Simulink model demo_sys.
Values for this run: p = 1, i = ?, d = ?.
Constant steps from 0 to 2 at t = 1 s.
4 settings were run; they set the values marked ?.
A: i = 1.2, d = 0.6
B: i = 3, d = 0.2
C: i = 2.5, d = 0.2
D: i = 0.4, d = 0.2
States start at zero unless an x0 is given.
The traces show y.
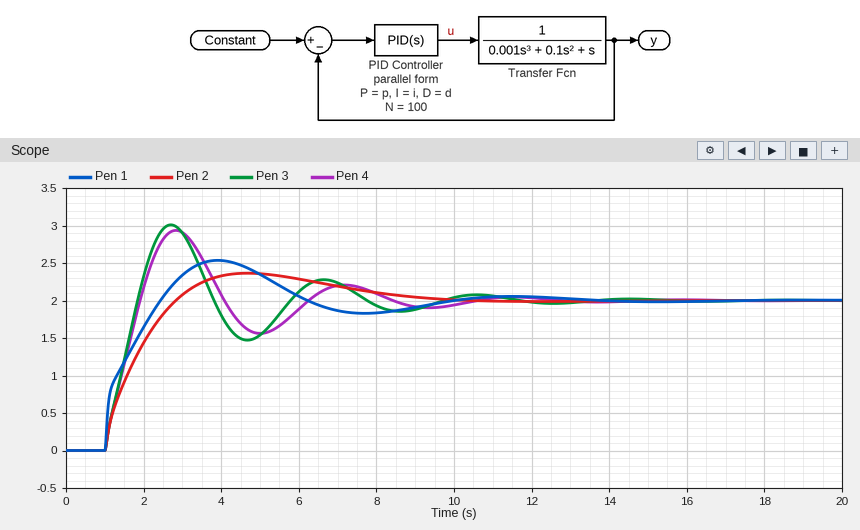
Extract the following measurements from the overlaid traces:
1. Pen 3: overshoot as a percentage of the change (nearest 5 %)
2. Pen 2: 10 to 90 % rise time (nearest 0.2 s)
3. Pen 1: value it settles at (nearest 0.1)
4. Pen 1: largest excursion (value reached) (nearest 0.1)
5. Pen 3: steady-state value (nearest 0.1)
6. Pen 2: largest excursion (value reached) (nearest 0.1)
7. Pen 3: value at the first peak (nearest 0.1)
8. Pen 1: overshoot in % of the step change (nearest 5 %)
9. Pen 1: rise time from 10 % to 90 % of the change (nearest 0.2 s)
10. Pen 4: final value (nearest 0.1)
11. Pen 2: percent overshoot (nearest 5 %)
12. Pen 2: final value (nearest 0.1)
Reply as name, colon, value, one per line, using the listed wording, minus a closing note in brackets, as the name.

Pen 3: overshoot as a percentage of the change: 50 %
Pen 2: 10 to 90 % rise time: 1.4 s
Pen 1: value it settles at: 2.0
Pen 1: largest excursion (value reached): 2.5
Pen 3: steady-state value: 2.0
Pen 2: largest excursion (value reached): 2.4
Pen 3: value at the first peak: 3.0
Pen 1: overshoot in % of the step change: 25 %
Pen 1: rise time from 10 % to 90 % of the change: 1.2 s
Pen 4: final value: 2.0
Pen 2: percent overshoot: 20 %
Pen 2: final value: 2.0
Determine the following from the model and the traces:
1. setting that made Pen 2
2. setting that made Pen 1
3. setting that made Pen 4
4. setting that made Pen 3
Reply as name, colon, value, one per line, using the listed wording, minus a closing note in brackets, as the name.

setting that made Pen 2: D
setting that made Pen 1: A
setting that made Pen 4: C
setting that made Pen 3: B
